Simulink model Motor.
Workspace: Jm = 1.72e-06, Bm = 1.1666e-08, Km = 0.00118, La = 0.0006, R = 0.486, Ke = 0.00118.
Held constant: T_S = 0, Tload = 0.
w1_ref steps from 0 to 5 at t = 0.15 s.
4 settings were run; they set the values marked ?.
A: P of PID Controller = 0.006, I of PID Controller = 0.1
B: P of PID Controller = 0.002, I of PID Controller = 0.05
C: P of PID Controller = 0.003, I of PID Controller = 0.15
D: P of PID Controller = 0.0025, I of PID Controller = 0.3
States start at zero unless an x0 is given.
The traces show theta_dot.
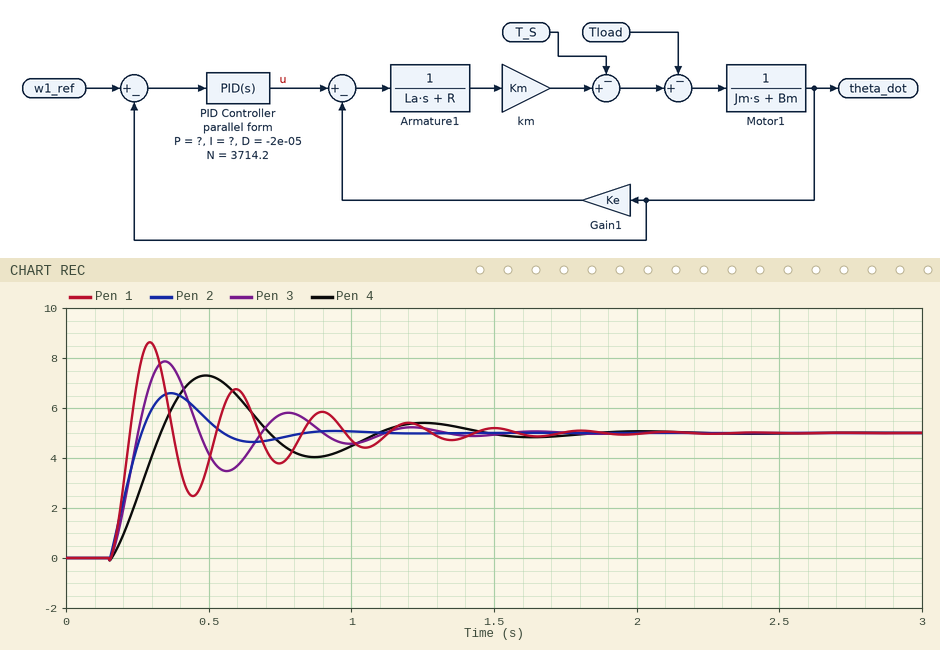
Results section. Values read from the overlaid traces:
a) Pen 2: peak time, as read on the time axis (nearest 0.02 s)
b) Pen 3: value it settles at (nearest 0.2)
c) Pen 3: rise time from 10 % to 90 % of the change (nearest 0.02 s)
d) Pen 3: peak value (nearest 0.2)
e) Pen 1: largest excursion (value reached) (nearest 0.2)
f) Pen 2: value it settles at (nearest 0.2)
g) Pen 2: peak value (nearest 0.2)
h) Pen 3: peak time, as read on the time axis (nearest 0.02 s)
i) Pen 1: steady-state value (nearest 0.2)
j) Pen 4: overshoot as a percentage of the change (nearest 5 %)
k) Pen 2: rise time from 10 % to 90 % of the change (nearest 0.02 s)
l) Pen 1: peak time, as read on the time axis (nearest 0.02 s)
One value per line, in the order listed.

0.36 s
5.0
0.08 s
7.8
8.6
5.0
6.6
0.34 s
5.0
45 %
0.08 s
0.30 s
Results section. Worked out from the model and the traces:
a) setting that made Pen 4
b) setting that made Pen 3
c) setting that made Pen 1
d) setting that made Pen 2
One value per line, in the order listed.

B
C
D
A
